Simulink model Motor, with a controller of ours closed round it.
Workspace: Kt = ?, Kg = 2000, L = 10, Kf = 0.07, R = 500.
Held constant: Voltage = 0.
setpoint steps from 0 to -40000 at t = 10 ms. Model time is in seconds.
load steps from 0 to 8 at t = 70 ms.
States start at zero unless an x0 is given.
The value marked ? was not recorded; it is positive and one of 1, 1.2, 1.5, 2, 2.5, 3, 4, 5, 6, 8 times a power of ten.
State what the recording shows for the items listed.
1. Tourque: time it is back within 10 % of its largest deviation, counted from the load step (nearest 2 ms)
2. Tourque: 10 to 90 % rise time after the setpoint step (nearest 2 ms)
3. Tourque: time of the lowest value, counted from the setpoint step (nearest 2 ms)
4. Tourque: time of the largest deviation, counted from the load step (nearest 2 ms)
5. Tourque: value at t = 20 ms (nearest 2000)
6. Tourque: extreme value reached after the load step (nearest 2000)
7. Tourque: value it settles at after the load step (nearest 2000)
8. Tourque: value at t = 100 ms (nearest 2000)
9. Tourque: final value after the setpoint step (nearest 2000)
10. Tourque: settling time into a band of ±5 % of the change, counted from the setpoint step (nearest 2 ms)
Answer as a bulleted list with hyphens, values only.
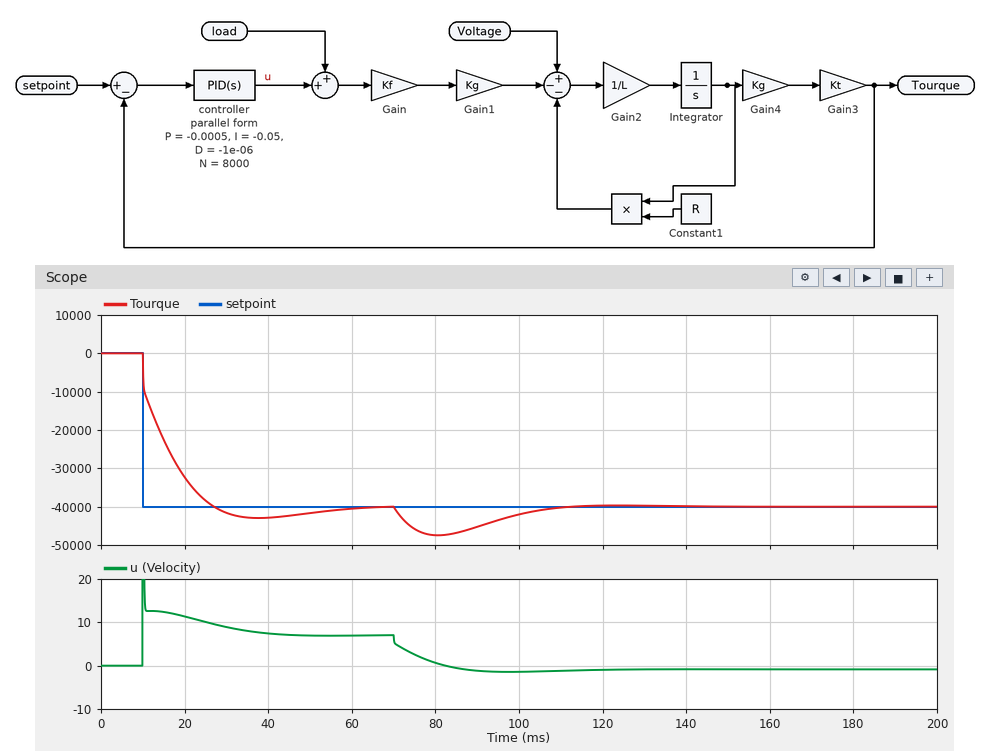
- 36 ms
- 12 ms
- 28 ms
- 10 ms
- -32000
- -48000
- -40000
- -42000
- -40000
- 38 ms
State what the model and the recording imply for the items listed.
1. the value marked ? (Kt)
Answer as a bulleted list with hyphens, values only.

- 10
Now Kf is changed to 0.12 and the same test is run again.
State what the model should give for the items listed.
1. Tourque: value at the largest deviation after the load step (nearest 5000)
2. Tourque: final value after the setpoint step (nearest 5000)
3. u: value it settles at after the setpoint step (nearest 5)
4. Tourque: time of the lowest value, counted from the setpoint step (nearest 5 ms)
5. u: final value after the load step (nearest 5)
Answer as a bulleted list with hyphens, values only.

- -50000
- -40000
- 5
- 20 ms
- -5
